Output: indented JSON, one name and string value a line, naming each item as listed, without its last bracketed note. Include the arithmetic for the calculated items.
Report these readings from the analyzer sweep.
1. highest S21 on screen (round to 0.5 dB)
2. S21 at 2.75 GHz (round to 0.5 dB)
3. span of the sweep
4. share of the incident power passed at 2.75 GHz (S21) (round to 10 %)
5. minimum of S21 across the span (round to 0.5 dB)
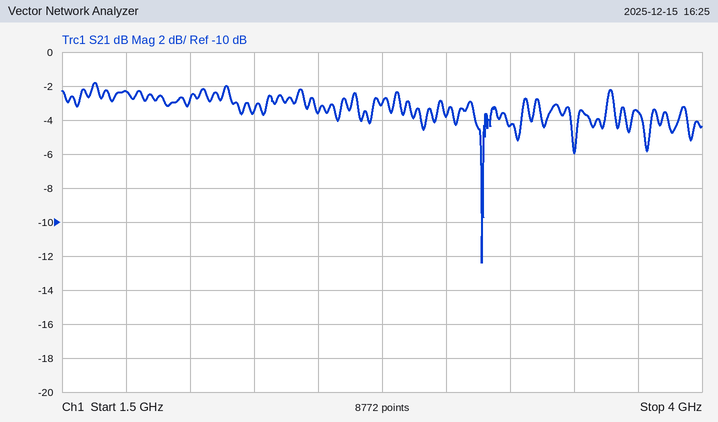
{
  "highest S21 on screen": "-2.0 dB",
  "S21 at 2.75 GHz": "-3.0 dB",
  "span of the sweep": "2.5 GHz",
  "share of the incident power passed at 2.75 GHz (S21)": "10^(-3/10) ≈ 50 %",
  "minimum of S21 across the span": "-12.5 dB"
}
